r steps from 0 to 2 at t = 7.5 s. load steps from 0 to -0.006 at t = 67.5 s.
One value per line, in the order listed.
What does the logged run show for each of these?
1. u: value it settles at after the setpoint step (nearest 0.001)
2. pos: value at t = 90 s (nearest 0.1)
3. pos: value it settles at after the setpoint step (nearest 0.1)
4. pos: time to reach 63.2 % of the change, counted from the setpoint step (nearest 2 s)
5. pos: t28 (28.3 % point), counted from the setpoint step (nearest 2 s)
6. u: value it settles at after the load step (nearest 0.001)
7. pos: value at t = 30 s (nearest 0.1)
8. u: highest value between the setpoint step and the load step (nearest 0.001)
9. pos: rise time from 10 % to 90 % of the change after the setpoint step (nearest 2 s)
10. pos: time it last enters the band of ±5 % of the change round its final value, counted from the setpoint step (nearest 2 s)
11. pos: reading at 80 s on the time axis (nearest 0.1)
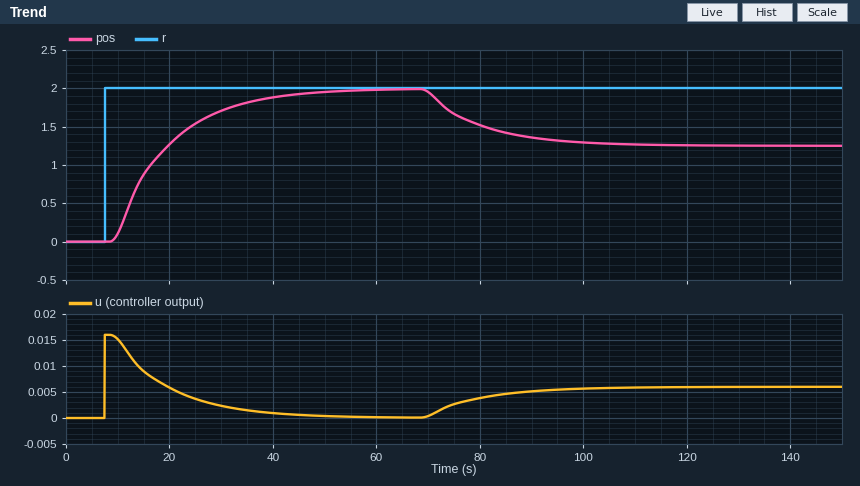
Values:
0.000
1.4
2.0
12 s
6 s
0.006
1.7
0.016
24 s
34 s
1.5
